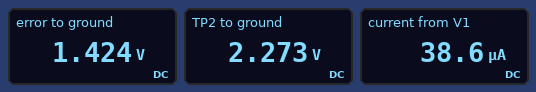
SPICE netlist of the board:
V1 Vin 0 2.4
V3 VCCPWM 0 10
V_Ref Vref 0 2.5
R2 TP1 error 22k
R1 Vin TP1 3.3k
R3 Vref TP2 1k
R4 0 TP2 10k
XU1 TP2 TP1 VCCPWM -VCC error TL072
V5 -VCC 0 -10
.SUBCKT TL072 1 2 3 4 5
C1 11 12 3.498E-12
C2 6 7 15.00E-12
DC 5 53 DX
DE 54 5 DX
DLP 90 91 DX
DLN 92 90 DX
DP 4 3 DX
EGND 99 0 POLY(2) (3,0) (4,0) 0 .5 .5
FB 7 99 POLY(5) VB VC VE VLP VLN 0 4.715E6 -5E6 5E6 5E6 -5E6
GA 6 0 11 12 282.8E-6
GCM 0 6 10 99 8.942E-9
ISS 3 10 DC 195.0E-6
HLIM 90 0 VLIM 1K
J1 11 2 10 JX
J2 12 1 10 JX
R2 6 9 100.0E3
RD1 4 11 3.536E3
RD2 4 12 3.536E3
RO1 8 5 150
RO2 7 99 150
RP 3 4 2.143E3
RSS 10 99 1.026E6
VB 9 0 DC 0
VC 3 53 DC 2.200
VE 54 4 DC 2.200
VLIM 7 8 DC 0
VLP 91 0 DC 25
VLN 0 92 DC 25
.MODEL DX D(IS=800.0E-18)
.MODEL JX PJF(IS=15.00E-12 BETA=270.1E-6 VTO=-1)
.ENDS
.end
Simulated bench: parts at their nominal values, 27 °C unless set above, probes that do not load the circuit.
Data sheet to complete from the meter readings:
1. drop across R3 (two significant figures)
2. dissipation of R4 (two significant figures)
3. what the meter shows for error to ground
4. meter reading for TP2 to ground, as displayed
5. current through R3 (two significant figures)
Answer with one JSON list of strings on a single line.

["230 mV", "520 µW", "1.424 V", "2.273 V", "230 µA"]
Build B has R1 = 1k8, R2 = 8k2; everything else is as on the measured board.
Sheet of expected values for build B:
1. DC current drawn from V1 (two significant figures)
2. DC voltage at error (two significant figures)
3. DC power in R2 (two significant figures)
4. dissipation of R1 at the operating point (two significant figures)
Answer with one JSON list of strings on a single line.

["71 µA", "1.7 V", "41 µW", "9.0 µW"]
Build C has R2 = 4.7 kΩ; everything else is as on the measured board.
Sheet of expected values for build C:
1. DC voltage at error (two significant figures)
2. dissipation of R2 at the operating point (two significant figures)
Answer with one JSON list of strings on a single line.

["2.1 V", "7.0 µW"]
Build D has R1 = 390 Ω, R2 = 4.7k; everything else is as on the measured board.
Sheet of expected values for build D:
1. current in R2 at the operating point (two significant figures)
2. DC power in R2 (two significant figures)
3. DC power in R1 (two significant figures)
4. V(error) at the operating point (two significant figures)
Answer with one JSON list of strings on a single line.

["330 µA", "500 µW", "42 µW", "740 mV"]
